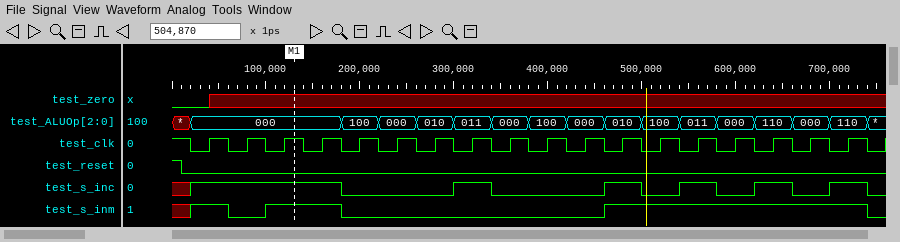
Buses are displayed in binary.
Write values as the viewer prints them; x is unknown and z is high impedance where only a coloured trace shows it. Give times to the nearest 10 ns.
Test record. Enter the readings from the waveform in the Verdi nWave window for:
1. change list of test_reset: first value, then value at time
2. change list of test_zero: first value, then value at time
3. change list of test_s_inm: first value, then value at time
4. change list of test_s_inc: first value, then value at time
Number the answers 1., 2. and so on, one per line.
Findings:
1. 1, 0 at 10 ns
2. 0, x at 40 ns
3. x, 1 at 20 ns, 0 at 60 ns, 1 at 100 ns, 0 at 180 ns, 1 at 460 ns, 0 at 740 ns
4. x, 1 at 20 ns, 0 at 180 ns, 1 at 300 ns, 0 at 340 ns, 1 at 460 ns, 0 at 500 ns, 1 at 540 ns, 0 at 580 ns, 1 at 620 ns, 0 at 660 ns, 1 at 700 ns, 0 at 740 ns
